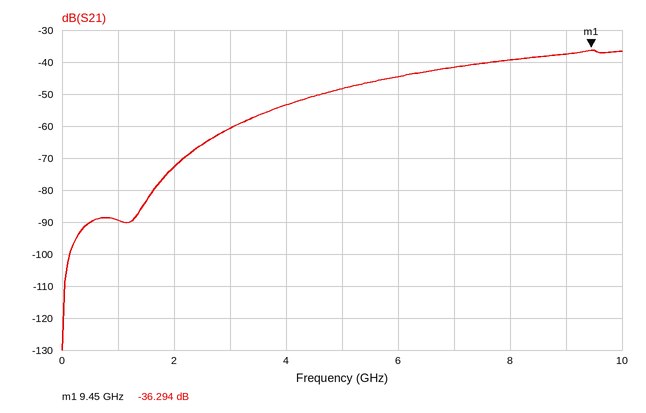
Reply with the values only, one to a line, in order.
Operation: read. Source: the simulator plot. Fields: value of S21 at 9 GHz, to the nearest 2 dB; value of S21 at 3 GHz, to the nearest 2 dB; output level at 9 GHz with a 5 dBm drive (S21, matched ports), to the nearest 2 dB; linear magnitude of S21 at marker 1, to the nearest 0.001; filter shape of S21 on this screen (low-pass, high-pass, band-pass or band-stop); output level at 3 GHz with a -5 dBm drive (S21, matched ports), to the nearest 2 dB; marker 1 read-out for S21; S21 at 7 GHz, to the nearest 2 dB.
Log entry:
-38 dB
-60 dB
-32 dBm
0.015
high-pass
-66 dBm
-36.294 dB
-42 dB
